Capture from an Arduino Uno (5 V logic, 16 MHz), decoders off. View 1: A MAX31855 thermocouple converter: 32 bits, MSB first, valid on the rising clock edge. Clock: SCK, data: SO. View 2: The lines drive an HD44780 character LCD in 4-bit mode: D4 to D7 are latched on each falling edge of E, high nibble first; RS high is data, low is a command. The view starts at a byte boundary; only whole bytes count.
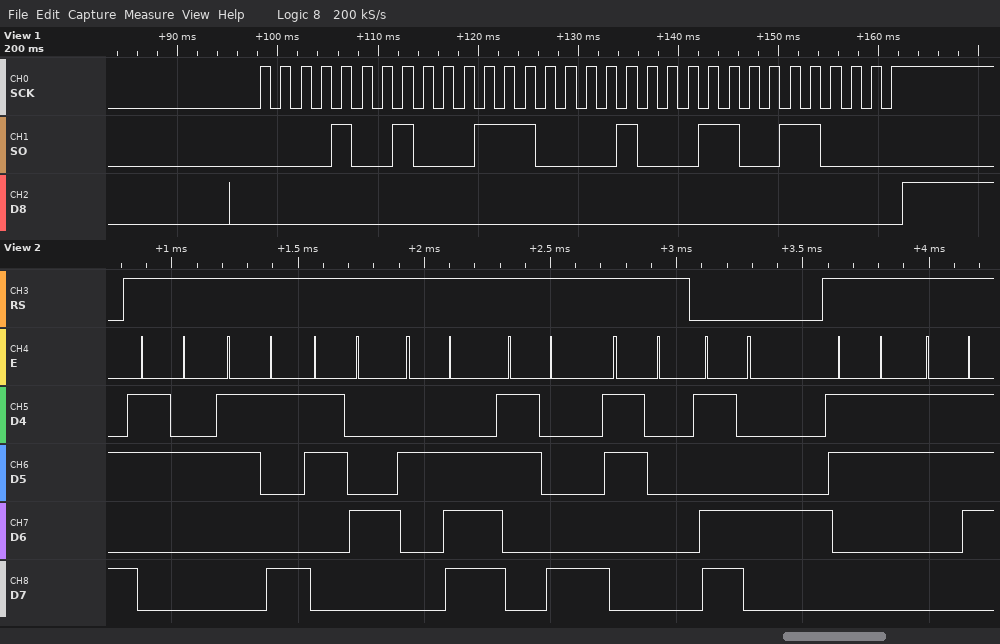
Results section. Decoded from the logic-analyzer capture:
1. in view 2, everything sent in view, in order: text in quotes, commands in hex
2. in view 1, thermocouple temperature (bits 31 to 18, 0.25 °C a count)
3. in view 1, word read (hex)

"294.80" 0xD4 "37"
145.75 °C
0x091C2330
